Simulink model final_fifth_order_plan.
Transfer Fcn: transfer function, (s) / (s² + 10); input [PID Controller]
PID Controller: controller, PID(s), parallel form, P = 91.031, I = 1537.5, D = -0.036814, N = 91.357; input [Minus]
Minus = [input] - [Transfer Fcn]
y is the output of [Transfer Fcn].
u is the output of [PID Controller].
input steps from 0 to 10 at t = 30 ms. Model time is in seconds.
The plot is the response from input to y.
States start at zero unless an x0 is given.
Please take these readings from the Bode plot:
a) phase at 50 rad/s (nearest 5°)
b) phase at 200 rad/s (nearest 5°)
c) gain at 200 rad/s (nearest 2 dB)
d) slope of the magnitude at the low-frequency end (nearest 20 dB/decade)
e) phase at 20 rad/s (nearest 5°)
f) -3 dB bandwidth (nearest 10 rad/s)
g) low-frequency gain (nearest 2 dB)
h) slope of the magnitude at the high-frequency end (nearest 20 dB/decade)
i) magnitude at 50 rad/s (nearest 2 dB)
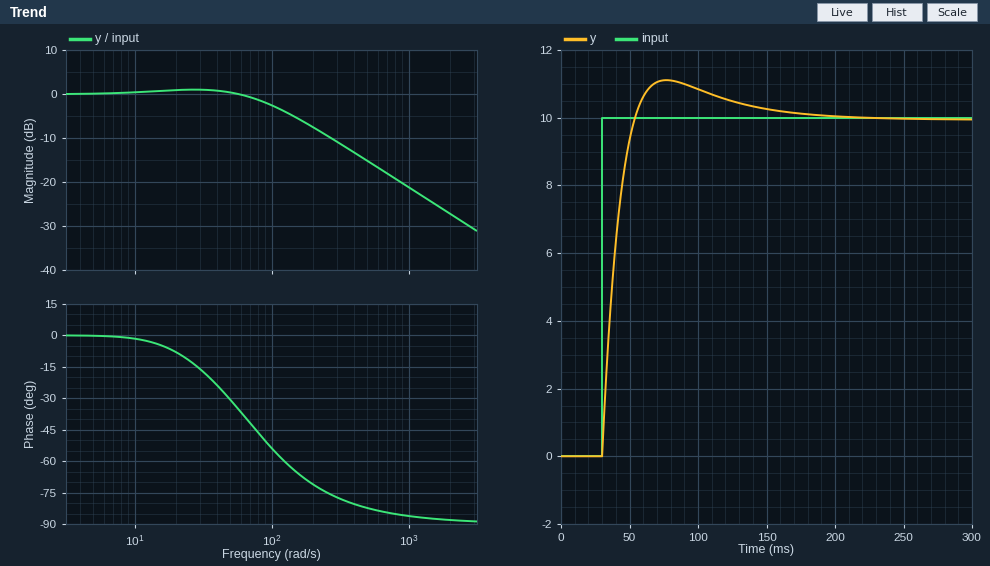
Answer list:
-30°
-70°
-8 dB
0 dB/decade
-10°
110 rad/s
0 dB
-20 dB/decade
0 dB
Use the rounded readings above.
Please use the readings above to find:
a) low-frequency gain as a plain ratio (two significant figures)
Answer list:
1.0
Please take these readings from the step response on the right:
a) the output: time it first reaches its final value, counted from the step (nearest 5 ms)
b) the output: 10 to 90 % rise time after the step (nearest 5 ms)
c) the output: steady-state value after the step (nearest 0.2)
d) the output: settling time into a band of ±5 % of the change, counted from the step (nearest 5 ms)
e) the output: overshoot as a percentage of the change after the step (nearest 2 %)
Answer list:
25 ms
15 ms
10.0
100 ms
12 %
